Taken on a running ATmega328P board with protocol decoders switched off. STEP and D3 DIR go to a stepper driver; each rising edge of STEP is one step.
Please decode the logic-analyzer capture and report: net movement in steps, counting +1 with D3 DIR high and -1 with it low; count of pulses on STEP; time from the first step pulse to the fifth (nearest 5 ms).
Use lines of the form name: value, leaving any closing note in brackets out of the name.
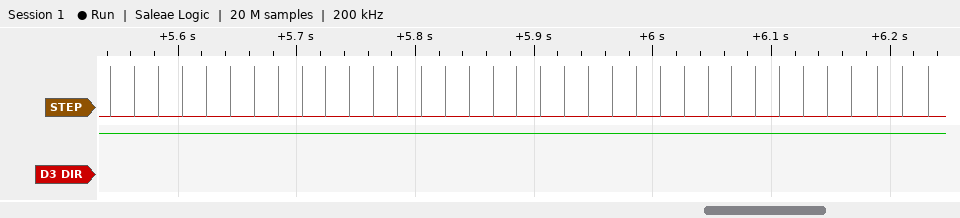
net movement in steps, counting +1 with D3 DIR high and -1 with it low: +35
count of pulses on STEP: 35
time from the first step pulse to the fifth: 80 ms
